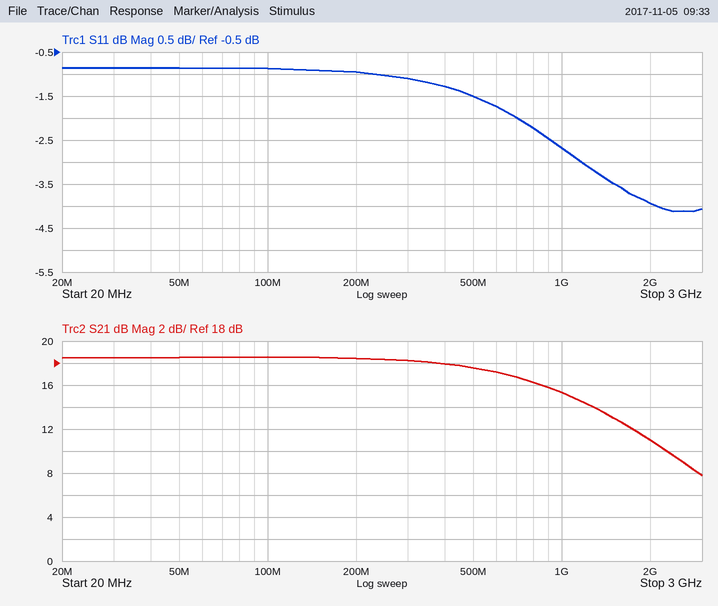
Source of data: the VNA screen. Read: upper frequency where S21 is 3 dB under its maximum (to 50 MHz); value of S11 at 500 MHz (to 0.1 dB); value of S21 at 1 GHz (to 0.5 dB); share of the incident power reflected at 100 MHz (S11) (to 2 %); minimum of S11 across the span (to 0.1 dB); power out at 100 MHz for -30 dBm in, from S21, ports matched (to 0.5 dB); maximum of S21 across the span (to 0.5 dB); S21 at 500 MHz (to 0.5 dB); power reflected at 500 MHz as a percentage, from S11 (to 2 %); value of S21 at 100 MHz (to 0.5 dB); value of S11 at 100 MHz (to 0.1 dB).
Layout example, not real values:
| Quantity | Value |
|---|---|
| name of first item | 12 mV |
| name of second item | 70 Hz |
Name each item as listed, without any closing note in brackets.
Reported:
| Quantity | Value |
|---|---|
| upper frequency where S21 is 3 dB under its maximum | 950 MHz |
| value of S11 at 500 MHz | -1.5 dB |
| value of S21 at 1 GHz | 15.5 dB |
| share of the incident power reflected at 100 MHz (S11) | 82 % |
| minimum of S11 across the span | -4.1 dB |
| power out at 100 MHz for -30 dBm in, from S21, ports matched | -11.5 dBm |
| maximum of S21 across the span | 18.5 dB |
| S21 at 500 MHz | 17.5 dB |
| power reflected at 500 MHz as a percentage, from S11 | 70 % |
| value of S21 at 100 MHz | 18.5 dB |
| value of S11 at 100 MHz | -0.9 dB |
